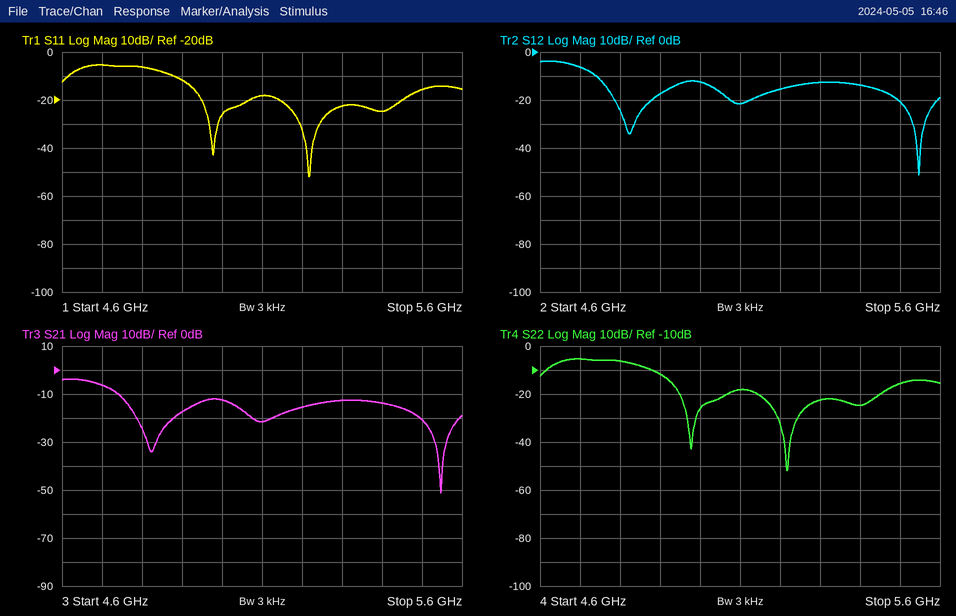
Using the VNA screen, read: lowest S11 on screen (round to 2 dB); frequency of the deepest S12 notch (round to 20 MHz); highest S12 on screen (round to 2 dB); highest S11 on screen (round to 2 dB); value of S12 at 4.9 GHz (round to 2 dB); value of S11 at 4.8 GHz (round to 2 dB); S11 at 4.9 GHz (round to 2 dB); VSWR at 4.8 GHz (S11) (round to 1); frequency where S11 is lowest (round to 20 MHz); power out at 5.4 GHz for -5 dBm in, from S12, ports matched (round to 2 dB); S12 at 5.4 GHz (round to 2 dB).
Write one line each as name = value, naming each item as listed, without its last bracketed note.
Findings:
lowest S11 on screen = -52 dB
frequency of the deepest S12 notch = 5.54 GHz
highest S12 on screen = -4 dB
highest S11 on screen = -6 dB
value of S12 at 4.9 GHz = -18 dB
value of S11 at 4.8 GHz = -6 dB
S11 at 4.9 GHz = -12 dB
VSWR at 4.8 GHz (S11) = 3
frequency where S11 is lowest = 5.22 GHz
power out at 5.4 GHz for -5 dBm in, from S12, ports matched = -18 dBm
S12 at 5.4 GHz = -14 dB
